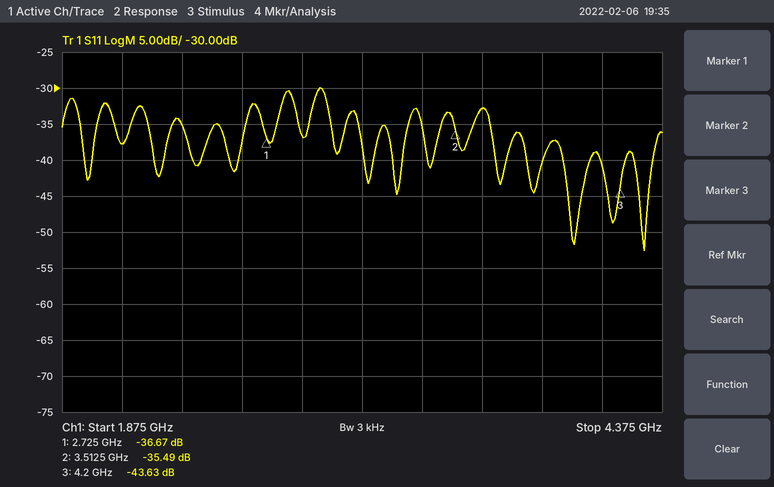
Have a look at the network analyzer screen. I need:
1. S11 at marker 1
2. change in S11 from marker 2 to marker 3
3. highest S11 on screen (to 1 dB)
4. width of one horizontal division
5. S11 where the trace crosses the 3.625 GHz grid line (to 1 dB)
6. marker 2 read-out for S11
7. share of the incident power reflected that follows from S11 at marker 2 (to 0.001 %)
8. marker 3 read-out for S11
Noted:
-36.67 dB
-8.14 dB
-30 dB
250 MHz
-33 dB
-35.49 dB
0.028 %
-43.63 dB
